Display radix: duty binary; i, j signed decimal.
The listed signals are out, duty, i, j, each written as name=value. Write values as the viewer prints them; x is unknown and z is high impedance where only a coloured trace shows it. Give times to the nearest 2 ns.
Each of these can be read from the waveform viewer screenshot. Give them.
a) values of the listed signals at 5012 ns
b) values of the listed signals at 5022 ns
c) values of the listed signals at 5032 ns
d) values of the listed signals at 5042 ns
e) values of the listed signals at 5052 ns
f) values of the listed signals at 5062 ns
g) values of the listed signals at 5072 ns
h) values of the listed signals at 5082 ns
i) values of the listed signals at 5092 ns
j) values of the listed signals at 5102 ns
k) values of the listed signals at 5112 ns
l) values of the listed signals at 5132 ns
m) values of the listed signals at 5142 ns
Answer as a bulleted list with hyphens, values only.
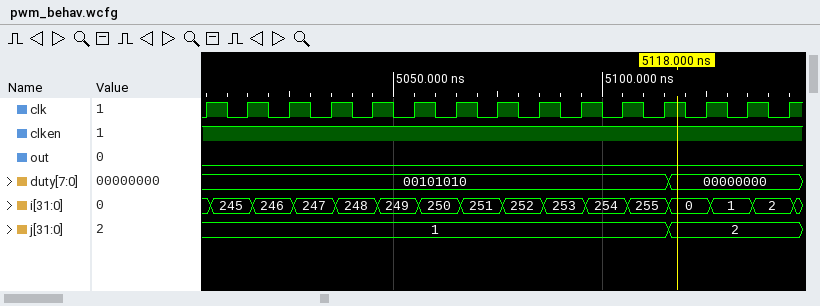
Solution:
- out=0, duty=00101010, i=245, j=1
- out=0, duty=00101010, i=246, j=1
- out=0, duty=00101010, i=247, j=1
- out=0, duty=00101010, i=248, j=1
- out=0, duty=00101010, i=249, j=1
- out=0, duty=00101010, i=250, j=1
- out=0, duty=00101010, i=251, j=1
- out=0, duty=00101010, i=252, j=1
- out=0, duty=00101010, i=253, j=1
- out=0, duty=00101010, i=254, j=1
- out=0, duty=00101010, i=255, j=1
- out=0, duty=00000000, i=1, j=2
- out=0, duty=00000000, i=2, j=2
